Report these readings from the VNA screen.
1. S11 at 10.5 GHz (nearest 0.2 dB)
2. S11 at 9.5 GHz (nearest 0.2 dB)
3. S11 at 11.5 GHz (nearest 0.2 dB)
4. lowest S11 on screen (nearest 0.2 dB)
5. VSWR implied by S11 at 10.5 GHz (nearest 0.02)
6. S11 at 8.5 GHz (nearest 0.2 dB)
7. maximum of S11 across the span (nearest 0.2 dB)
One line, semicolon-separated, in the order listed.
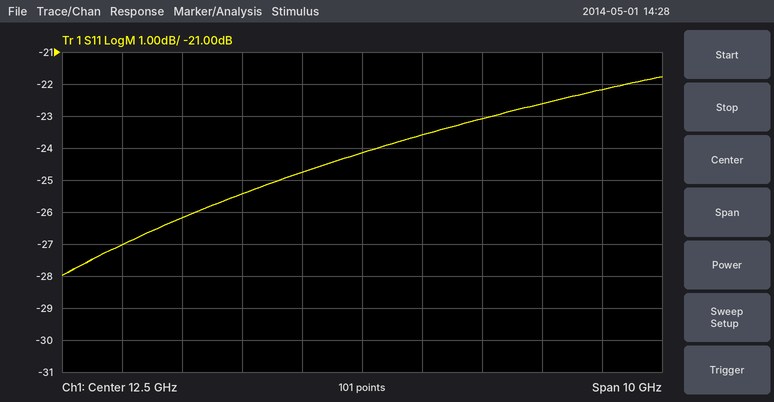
-25.4 dB; -26.2 dB; -24.8 dB; -28.0 dB; 1.12; -27.0 dB; -21.8 dB
